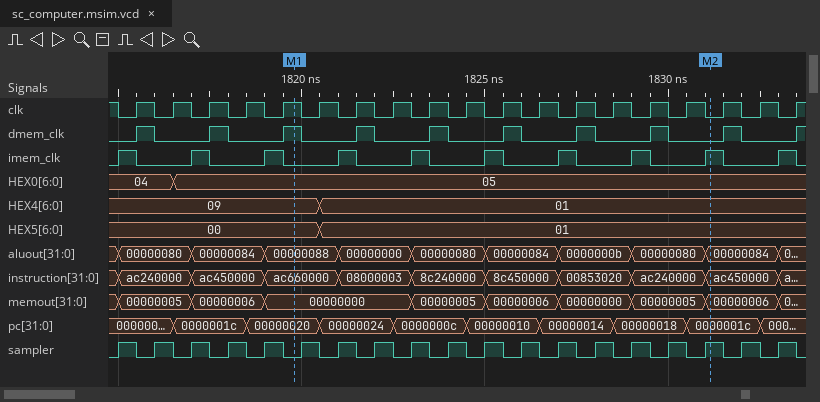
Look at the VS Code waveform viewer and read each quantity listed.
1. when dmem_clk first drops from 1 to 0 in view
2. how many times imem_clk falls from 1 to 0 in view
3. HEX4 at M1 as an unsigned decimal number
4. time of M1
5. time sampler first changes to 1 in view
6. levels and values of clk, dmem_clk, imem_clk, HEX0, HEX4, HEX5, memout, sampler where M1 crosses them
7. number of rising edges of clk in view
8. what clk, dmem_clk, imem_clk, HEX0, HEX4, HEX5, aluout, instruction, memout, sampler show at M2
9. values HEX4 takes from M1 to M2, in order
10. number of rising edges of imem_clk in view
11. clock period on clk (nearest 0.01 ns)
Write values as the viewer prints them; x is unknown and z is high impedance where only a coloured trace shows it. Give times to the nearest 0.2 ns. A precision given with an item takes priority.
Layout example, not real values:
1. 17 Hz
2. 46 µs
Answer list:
1. 1816 ns
2. 10
3. 9
4. 1819.8 ns
5. 1815 ns
6. clk=1, dmem_clk=1, imem_clk=0, HEX0=05, HEX4=09, HEX5=00, memout=00000000, sampler=0
7. 19
8. clk=0, dmem_clk=0, imem_clk=1, HEX0=05, HEX4=01, HEX5=01, aluout=00000084, instruction=ac450000, memout=00000006, sampler=1
9. 09, 01
10. 10
11. 1 ns
